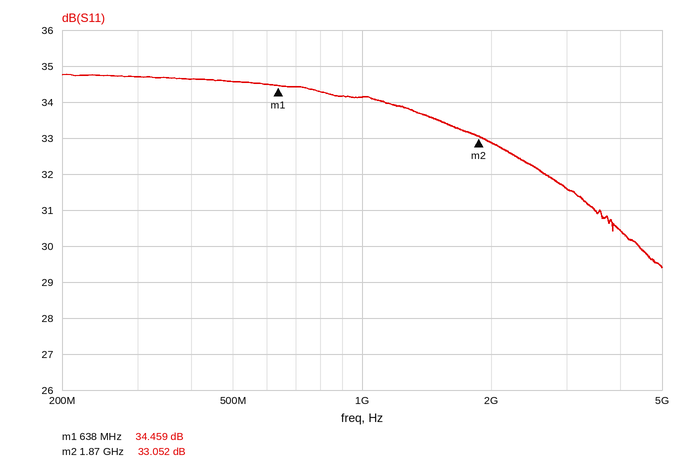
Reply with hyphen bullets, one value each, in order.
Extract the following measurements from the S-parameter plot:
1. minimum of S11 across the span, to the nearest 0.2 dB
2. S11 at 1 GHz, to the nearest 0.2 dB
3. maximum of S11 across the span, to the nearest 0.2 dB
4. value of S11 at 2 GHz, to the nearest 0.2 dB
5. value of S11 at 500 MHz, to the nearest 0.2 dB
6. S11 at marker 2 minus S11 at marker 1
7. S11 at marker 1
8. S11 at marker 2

- 29.4 dB
- 34.2 dB
- 34.8 dB
- 32.8 dB
- 34.6 dB
- -1.407 dB
- 34.459 dB
- 33.052 dB
